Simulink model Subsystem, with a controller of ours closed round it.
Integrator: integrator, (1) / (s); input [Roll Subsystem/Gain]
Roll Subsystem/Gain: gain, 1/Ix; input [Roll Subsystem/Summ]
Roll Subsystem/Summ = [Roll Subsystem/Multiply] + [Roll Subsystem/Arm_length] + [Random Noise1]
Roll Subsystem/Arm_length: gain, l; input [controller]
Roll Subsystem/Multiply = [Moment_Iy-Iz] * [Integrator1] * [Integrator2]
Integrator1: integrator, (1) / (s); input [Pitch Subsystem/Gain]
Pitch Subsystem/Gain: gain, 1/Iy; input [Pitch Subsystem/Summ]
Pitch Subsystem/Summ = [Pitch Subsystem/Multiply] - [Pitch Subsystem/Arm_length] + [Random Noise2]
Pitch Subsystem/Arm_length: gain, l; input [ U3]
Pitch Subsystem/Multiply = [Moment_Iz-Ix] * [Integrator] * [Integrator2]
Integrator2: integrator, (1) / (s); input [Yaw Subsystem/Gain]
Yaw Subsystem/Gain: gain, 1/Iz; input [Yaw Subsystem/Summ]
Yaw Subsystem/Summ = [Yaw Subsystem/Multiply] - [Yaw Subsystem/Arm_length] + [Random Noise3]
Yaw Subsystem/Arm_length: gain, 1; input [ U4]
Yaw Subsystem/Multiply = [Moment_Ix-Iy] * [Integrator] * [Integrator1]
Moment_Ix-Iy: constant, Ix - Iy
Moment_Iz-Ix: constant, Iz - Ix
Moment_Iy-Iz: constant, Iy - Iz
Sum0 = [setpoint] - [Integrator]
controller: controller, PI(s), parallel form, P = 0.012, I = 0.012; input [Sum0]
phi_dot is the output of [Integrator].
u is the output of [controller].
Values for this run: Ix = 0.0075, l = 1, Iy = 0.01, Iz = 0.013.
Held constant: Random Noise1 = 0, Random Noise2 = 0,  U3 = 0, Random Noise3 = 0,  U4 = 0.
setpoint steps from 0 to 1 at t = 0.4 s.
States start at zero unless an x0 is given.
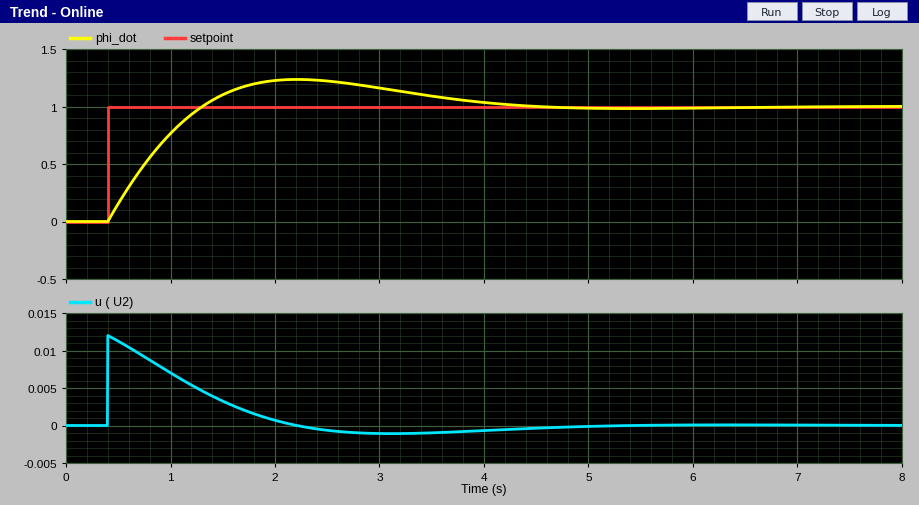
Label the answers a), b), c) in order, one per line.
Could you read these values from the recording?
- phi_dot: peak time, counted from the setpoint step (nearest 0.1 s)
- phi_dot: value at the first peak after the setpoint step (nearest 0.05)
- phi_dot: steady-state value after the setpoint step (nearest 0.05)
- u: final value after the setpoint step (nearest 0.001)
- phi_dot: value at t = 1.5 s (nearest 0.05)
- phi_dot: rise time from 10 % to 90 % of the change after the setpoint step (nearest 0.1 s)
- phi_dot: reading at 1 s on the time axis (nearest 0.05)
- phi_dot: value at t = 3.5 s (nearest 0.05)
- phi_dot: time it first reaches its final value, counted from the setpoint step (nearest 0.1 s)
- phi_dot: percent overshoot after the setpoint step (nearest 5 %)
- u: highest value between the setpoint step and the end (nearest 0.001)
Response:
a) 1.8 s
b) 1.25
c) 1.00
d) 0.000
e) 1.10
f) 0.7 s
g) 0.75
h) 1.10
i) 0.9 s
j) 25 %
k) 0.012
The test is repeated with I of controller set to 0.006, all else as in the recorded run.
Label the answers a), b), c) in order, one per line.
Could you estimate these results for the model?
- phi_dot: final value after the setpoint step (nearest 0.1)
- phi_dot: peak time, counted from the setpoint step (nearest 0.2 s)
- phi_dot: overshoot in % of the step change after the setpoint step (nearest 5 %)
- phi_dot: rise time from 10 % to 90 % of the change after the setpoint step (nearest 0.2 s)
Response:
a) 1.0
b) 2.4 s
c) 15 %
d) 0.8 s
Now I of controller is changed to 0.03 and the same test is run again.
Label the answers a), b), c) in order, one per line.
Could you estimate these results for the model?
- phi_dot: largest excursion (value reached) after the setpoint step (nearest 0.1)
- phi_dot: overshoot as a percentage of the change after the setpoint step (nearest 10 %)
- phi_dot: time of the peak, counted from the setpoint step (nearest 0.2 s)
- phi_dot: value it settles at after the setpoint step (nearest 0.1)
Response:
a) 1.4
b) 40 %
c) 1.2 s
d) 1.0
